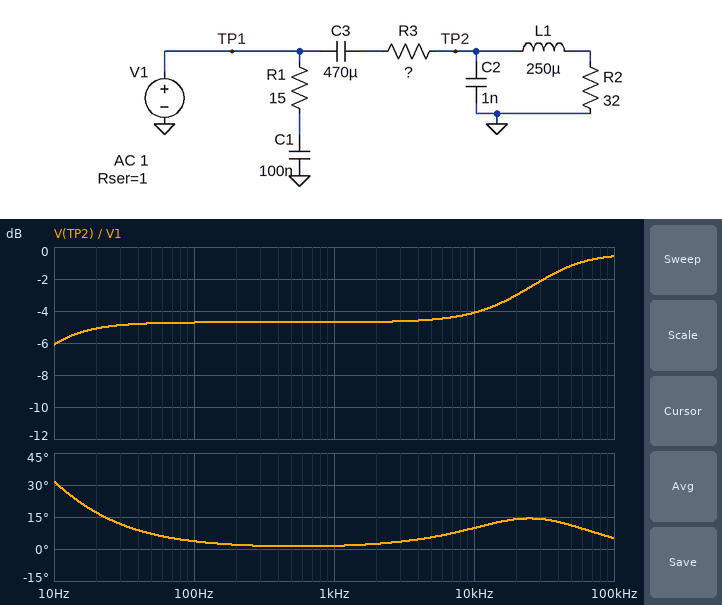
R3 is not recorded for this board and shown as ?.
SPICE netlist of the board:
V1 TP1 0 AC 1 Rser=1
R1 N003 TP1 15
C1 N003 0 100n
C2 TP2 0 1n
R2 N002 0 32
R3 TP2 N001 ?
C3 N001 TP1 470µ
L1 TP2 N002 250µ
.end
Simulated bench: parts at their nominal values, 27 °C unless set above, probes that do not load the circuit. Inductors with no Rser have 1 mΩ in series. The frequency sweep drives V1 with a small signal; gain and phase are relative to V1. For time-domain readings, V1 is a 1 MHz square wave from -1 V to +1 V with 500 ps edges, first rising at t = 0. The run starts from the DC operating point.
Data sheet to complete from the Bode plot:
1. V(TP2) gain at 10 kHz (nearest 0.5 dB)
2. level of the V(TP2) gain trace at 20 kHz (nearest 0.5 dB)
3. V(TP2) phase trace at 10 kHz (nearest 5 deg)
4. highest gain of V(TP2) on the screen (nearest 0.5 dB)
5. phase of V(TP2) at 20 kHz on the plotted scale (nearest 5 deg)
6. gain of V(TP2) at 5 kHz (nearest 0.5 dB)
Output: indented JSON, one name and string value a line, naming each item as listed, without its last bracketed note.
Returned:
{
  "V(TP2) gain at 10 kHz": "-4.0 dB",
  "level of the V(TP2) gain trace at 20 kHz": "-3.0 dB",
  "V(TP2) phase trace at 10 kHz": "10 deg",
  "highest gain of V(TP2) on the screen": "-0.5 dB",
  "phase of V(TP2) at 20 kHz on the plotted scale": "15 deg",
  "gain of V(TP2) at 5 kHz": "-4.5 dB"
}
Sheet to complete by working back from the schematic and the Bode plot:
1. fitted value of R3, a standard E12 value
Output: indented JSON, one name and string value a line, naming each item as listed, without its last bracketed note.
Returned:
{
  "fitted value of R3, a standard E12 value": "22 Ω"
}
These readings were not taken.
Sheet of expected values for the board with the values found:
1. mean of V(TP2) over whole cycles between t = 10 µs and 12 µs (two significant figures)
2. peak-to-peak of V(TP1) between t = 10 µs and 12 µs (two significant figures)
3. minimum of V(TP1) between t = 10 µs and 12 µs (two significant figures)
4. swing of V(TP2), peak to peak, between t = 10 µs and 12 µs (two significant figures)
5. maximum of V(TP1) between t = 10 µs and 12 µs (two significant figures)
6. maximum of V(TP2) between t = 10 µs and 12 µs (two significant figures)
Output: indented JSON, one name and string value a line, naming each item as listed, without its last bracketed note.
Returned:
{
  "mean of V(TP2) over whole cycles between t = 10 µs and 12 µs": "620 mV",
  "peak-to-peak of V(TP1) between t = 10 µs and 12 µs": "1.9 V",
  "minimum of V(TP1) between t = 10 µs and 12 µs": "-960 mV",
  "swing of V(TP2), peak to peak, between t = 10 µs and 12 µs": "1.9 V",
  "maximum of V(TP1) between t = 10 µs and 12 µs": "930 mV",
  "maximum of V(TP2) between t = 10 µs and 12 µs": "1.6 V"
}
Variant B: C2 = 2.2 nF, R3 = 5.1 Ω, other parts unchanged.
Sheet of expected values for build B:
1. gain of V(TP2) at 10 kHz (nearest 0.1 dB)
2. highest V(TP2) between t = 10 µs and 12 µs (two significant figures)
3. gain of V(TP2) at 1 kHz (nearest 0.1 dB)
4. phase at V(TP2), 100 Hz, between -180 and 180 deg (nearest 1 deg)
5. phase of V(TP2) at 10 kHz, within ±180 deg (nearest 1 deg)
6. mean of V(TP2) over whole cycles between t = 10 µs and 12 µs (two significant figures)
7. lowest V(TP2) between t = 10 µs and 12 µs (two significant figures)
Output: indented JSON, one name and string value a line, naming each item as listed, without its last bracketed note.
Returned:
{
  "gain of V(TP2) at 10 kHz": "-1.3 dB",
  "highest V(TP2) between t = 10 µs and 12 µs": "1.8 V",
  "gain of V(TP2) at 1 kHz": "-1.5 dB",
  "phase at V(TP2), 100 Hz, between -180 and 180 deg": "5 deg",
  "phase of V(TP2) at 10 kHz, within ±180 deg": "3 deg",
  "mean of V(TP2) over whole cycles between t = 10 µs and 12 µs": "870 mV",
  "lowest V(TP2) between t = 10 µs and 12 µs": "-77 mV"
}
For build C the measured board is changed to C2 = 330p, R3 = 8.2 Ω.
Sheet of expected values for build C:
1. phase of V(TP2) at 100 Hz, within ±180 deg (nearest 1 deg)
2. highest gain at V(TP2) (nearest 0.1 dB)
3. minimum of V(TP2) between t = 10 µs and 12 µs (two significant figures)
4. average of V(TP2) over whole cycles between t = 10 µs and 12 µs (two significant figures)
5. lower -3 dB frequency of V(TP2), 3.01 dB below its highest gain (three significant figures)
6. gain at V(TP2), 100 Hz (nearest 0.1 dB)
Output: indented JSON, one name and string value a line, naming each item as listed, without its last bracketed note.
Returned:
{
  "phase of V(TP2) at 100 Hz, within ±180 deg": "5 deg",
  "highest gain at V(TP2)": "-0.4 dB",
  "minimum of V(TP2) between t = 10 µs and 12 µs": "-130 mV",
  "average of V(TP2) over whole cycles between t = 10 µs and 12 µs": "810 mV",
  "lower -3 dB frequency of V(TP2), 3.01 dB below its highest gain": "14.6 Hz",
  "gain at V(TP2), 100 Hz": "-2.2 dB"
}
